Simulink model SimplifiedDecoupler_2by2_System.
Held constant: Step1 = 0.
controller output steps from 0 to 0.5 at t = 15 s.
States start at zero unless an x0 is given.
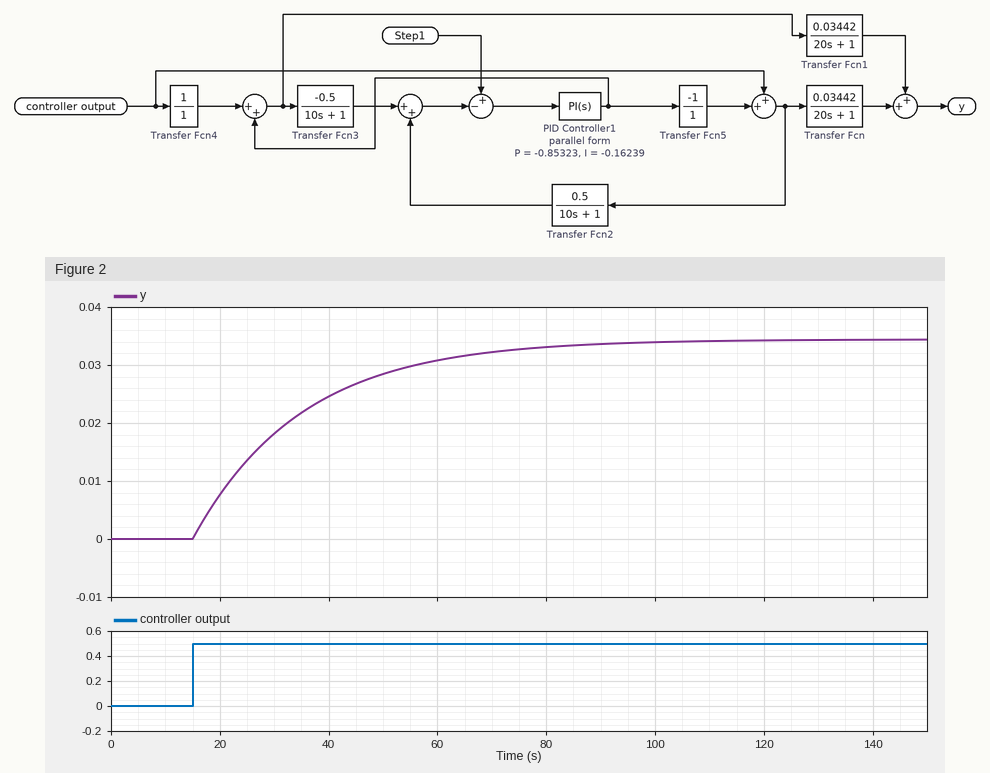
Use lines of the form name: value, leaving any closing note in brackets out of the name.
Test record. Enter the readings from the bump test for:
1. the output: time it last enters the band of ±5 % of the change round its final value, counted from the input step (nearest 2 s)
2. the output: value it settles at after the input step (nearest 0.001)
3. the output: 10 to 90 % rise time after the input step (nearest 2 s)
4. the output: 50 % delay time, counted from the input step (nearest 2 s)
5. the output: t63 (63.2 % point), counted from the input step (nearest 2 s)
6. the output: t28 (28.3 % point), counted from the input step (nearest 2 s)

the output: time it last enters the band of ±5 % of the change round its final value, counted from the input step: 60 s
the output: value it settles at after the input step: 0.034
the output: 10 to 90 % rise time after the input step: 44 s
the output: 50 % delay time, counted from the input step: 14 s
the output: t63 (63.2 % point), counted from the input step: 20 s
the output: t28 (28.3 % point), counted from the input step: 6 s
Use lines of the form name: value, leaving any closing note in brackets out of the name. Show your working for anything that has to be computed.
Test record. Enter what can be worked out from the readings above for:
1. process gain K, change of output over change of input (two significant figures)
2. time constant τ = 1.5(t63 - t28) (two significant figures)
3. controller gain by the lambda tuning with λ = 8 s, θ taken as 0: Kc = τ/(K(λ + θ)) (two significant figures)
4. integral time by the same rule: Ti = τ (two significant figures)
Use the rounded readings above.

process gain K, change of output over change of input: (0.034 - 0) / 0.5 = 0.068
time constant τ = 1.5(t63 - t28): 1.5 × (20 - 6) = 21 s
controller gain by the lambda tuning with λ = 8 s, θ taken as 0: Kc = τ/(K(λ + θ)): 21 / (0.068 × (8 + 0)) = 39
integral time by the same rule: Ti = τ: 21 s
